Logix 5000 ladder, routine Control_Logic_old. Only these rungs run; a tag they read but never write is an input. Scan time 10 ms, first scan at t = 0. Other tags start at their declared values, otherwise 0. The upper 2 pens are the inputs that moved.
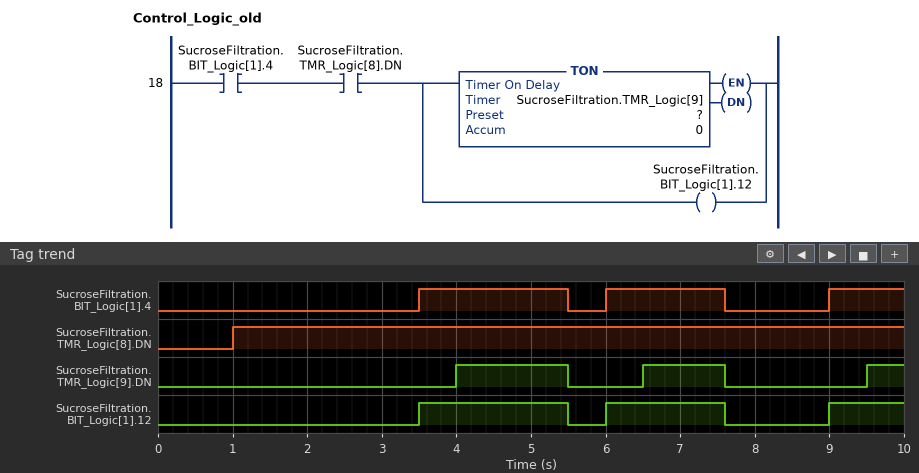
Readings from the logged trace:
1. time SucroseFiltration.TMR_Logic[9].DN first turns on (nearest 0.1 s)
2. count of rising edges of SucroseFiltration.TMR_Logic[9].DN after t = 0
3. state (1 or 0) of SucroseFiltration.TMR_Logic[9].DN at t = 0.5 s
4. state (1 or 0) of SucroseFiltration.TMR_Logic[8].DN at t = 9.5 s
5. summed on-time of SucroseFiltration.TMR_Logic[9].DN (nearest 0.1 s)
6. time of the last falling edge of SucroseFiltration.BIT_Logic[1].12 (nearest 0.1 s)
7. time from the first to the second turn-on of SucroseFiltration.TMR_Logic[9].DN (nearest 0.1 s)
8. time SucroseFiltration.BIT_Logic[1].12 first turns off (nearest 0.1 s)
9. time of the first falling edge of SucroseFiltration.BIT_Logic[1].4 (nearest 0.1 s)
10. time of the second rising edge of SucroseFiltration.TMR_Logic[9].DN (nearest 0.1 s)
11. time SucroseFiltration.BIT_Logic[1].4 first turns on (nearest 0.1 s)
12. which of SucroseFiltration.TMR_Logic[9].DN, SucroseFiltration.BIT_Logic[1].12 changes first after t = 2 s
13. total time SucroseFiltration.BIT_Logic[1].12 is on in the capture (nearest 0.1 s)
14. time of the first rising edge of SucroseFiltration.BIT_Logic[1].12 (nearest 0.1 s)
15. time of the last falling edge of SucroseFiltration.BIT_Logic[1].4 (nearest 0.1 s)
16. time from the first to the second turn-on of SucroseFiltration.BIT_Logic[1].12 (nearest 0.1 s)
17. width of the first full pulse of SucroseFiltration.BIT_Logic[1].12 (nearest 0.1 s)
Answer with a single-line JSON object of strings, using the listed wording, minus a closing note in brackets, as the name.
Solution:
{"time SucroseFiltration.TMR_Logic[9].DN first turns on": "4.0 s", "count of rising edges of SucroseFiltration.TMR_Logic[9].DN after t = 0": "3", "state (1 or 0) of SucroseFiltration.TMR_Logic[9].DN at t = 0.5 s": "0", "state (1 or 0) of SucroseFiltration.TMR_Logic[8].DN at t = 9.5 s": "1", "summed on-time of SucroseFiltration.TMR_Logic[9].DN": "3.1 s", "time of the last falling edge of SucroseFiltration.BIT_Logic[1].12": "7.6 s", "time from the first to the second turn-on of SucroseFiltration.TMR_Logic[9].DN": "2.5 s", "time SucroseFiltration.BIT_Logic[1].12 first turns off": "5.5 s", "time of the first falling edge of SucroseFiltration.BIT_Logic[1].4": "5.5 s", "time of the second rising edge of SucroseFiltration.TMR_Logic[9].DN": "6.5 s", "time SucroseFiltration.BIT_Logic[1].4 first turns on": "3.5 s", "which of SucroseFiltration.TMR_Logic[9].DN, SucroseFiltration.BIT_Logic[1].12 changes first after t = 2 s": "SucroseFiltration.BIT_Logic[1].12", "total time SucroseFiltration.BIT_Logic[1].12 is on in the capture": "4.6 s", "time of the first rising edge of SucroseFiltration.BIT_Logic[1].12": "3.5 s", "time of the last falling edge of SucroseFiltration.BIT_Logic[1].4": "7.6 s", "time from the first to the second turn-on of SucroseFiltration.BIT_Logic[1].12": "2.5 s", "width of the first full pulse of SucroseFiltration.BIT_Logic[1].12": "2.0 s"}
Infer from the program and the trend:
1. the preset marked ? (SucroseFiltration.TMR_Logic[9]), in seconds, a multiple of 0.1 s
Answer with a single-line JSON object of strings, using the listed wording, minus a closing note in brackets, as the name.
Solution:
{"the preset marked ? (SucroseFiltration.TMR_Logic[9]), in seconds, a multiple of 0.1 s": "0.5 s"}
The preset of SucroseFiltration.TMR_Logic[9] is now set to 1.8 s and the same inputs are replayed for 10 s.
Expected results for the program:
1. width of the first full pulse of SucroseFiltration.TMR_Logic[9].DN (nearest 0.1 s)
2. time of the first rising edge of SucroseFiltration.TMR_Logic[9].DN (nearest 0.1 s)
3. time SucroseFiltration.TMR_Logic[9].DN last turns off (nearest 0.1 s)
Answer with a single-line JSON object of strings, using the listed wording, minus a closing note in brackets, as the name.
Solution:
{"width of the first full pulse of SucroseFiltration.TMR_Logic[9].DN": "0.2 s", "time of the first rising edge of SucroseFiltration.TMR_Logic[9].DN": "5.3 s", "time SucroseFiltration.TMR_Logic[9].DN last turns off": "5.5 s"}
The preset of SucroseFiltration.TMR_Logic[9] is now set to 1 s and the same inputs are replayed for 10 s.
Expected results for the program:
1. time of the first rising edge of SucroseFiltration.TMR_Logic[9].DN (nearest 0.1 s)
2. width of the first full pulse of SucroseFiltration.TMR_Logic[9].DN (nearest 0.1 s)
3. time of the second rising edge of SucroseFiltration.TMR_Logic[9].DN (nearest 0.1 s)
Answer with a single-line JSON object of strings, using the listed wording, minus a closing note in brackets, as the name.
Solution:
{"time of the first rising edge of SucroseFiltration.TMR_Logic[9].DN": "4.5 s", "width of the first full pulse of SucroseFiltration.TMR_Logic[9].DN": "1.0 s", "time of the second rising edge of SucroseFiltration.TMR_Logic[9].DN": "7.0 s"}
